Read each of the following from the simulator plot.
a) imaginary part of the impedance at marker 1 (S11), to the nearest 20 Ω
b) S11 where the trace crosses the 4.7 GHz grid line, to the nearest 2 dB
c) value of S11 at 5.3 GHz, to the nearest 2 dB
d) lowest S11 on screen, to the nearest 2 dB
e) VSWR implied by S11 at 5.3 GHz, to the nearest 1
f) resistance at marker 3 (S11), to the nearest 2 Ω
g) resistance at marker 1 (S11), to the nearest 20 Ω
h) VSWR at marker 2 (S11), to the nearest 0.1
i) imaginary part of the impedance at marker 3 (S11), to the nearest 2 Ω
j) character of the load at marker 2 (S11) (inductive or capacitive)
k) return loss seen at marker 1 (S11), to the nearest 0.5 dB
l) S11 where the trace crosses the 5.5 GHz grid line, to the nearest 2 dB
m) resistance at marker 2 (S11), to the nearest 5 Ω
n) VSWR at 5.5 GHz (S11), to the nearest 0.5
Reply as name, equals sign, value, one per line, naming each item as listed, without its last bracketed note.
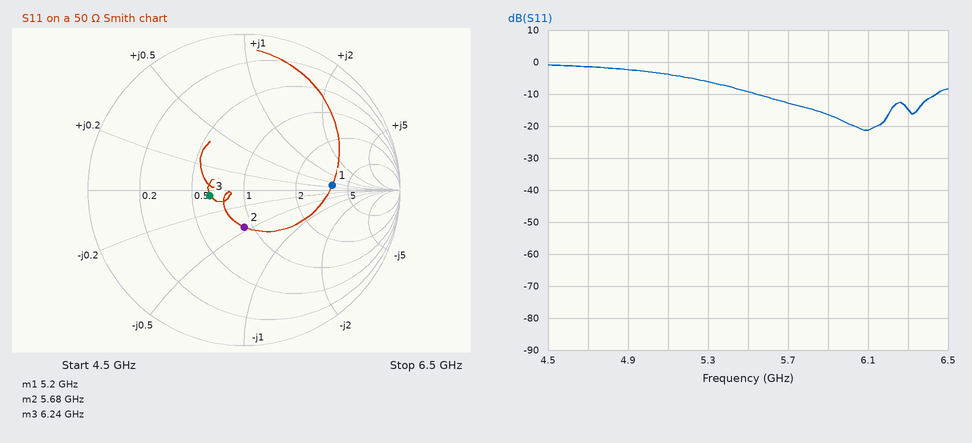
imaginary part of the impedance at marker 1 (S11), to the nearest 20 Ω = +20 Ω
S11 where the trace crosses the 4.7 GHz grid line, to the nearest 2 dB = -2 dB
value of S11 at 5.3 GHz, to the nearest 2 dB = -6 dB
lowest S11 on screen, to the nearest 2 dB = -22 dB
VSWR implied by S11 at 5.3 GHz, to the nearest 1 = 3
resistance at marker 3 (S11), to the nearest 2 Ω = 32 Ω
resistance at marker 1 (S11), to the nearest 20 Ω = 180 Ω
VSWR at marker 2 (S11), to the nearest 0.1 = 1.6
imaginary part of the impedance at marker 3 (S11), to the nearest 2 Ω = -2 Ω
character of the load at marker 2 (S11) = capacitive
return loss seen at marker 1 (S11), to the nearest 0.5 dB = 5.0 dB
S11 where the trace crosses the 5.5 GHz grid line, to the nearest 2 dB = -10 dB
resistance at marker 2 (S11), to the nearest 5 Ω = 45 Ω
VSWR at 5.5 GHz (S11), to the nearest 0.5 = 2.0
